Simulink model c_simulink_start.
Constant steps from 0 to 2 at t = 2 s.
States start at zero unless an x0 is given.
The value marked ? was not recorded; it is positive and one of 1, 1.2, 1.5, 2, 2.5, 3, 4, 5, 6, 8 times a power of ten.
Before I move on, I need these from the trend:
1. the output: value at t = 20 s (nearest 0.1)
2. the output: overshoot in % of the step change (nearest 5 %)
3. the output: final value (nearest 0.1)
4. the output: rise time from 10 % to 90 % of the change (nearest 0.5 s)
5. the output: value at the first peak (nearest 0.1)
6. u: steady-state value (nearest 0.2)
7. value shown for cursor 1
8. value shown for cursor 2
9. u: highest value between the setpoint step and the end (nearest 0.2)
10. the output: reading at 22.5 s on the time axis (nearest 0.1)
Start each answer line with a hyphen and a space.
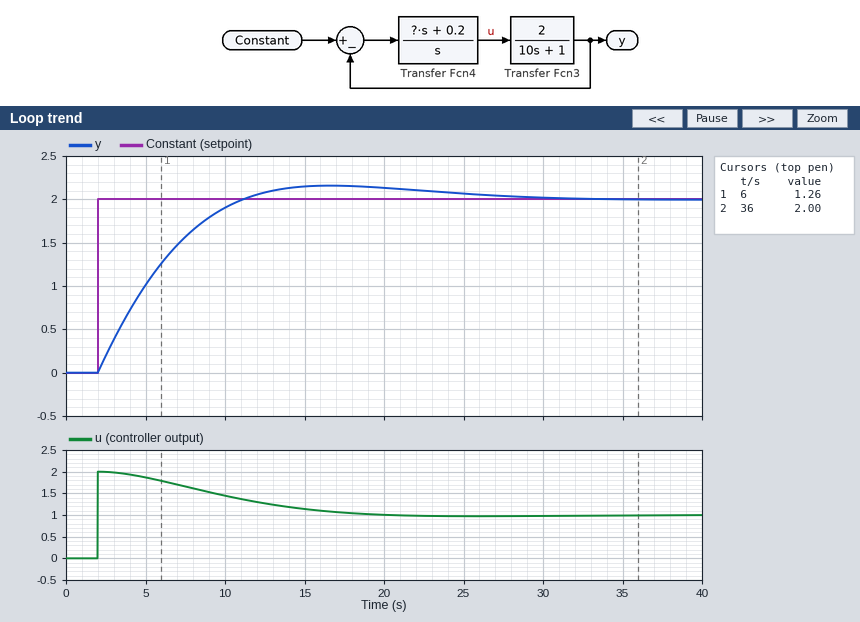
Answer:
- 2.1
- 10 %
- 2.0
- 6.5 s
- 2.2
- 1.0
- 1.26
- 2.00
- 2.0
- 2.1
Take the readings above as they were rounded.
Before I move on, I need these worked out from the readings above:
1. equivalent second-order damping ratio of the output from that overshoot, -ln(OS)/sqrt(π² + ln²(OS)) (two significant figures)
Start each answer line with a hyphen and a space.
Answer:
- 0.59
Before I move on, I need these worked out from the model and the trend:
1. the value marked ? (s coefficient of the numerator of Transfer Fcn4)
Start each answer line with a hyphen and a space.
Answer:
- 1
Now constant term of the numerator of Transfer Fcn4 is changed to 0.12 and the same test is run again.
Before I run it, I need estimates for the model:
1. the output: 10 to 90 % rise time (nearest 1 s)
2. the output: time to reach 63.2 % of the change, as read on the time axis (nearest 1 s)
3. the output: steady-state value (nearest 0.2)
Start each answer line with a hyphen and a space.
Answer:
- 9 s
- 7 s
- 2.0
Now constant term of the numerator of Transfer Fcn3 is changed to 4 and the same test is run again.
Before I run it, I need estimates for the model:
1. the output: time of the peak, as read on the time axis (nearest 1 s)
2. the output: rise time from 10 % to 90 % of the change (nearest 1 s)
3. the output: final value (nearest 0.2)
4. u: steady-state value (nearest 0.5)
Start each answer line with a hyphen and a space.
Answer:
- 11 s
- 4 s
- 2.0
- 0.5
